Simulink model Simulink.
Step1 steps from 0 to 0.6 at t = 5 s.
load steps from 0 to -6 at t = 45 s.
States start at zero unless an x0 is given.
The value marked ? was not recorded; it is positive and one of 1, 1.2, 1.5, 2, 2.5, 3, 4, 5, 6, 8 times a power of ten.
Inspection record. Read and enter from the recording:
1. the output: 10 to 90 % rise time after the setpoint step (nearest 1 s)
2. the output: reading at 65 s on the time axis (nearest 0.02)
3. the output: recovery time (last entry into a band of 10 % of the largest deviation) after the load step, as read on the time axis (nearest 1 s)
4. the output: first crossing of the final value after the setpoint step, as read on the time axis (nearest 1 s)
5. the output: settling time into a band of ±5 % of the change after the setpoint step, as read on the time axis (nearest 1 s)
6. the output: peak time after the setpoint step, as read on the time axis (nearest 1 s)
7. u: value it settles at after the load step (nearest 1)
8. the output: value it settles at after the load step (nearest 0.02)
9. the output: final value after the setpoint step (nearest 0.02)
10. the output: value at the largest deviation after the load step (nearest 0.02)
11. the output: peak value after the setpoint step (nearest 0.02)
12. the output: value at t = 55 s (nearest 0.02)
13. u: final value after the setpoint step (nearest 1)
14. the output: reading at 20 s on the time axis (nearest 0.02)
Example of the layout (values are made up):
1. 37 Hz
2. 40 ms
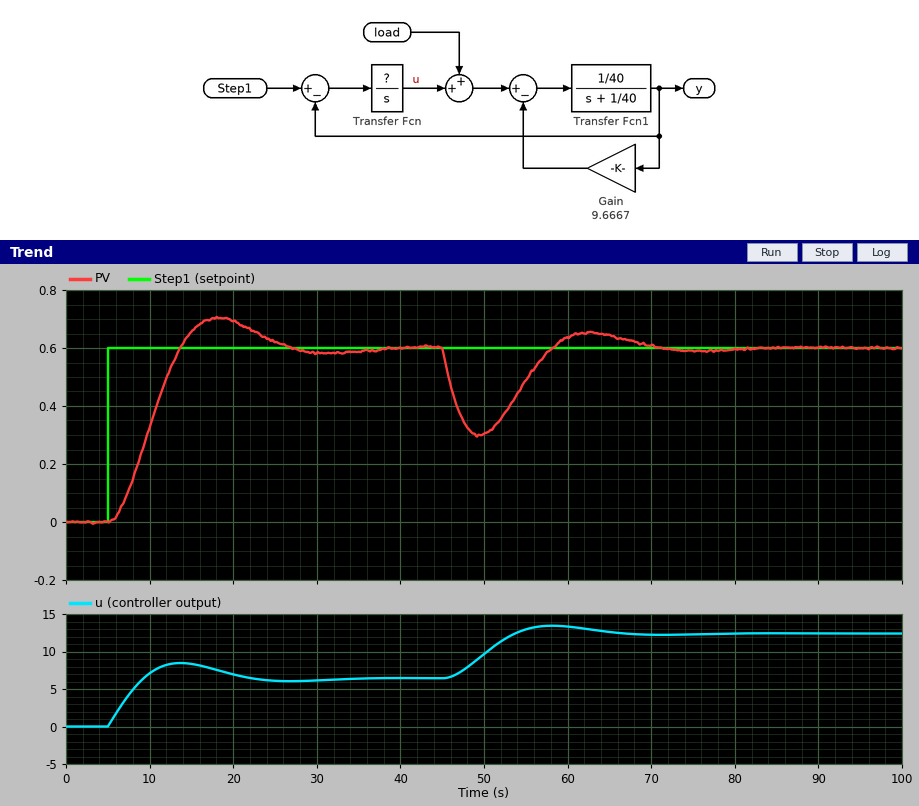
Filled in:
1. 6 s
2. 0.64
3. 67 s
4. 14 s
5. 24 s
6. 18 s
7. 12
8. 0.60
9. 0.60
10. 0.30
11. 0.70
12. 0.48
13. 6
14. 0.70
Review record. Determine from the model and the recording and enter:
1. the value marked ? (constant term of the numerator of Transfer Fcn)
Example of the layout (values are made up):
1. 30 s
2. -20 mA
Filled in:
1. 3
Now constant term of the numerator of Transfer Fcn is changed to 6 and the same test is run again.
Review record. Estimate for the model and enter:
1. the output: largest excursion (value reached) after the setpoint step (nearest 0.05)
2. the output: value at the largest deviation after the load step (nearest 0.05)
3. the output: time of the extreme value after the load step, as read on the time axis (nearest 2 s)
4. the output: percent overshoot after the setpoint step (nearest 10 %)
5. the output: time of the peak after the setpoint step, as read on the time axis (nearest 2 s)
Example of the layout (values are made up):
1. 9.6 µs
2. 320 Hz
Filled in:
1. 0.80
2. 0.35
3. 48 s
4. 30 %
5. 14 s
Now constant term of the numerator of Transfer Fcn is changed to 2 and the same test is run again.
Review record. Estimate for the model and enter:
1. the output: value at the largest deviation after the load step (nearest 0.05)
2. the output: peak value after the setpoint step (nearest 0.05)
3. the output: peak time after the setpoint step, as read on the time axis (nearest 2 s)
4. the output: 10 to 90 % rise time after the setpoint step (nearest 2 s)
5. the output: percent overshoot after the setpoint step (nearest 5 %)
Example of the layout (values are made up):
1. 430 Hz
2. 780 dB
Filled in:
1. 0.25
2. 0.65
3. 22 s
4. 8 s
5. 10 %
